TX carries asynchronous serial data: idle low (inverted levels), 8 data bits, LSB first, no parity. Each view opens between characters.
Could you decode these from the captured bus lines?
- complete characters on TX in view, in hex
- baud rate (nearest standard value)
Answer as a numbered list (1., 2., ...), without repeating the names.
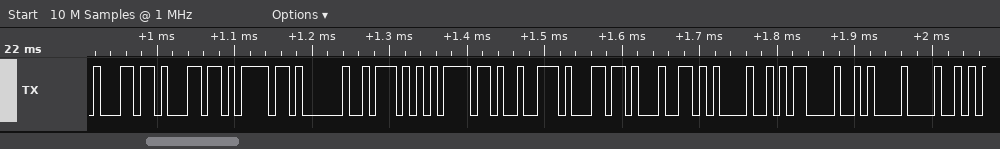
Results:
1. 27, 27, 21, BF, 51, 21, 1B, 27, 37, BD, E5, EB, 6F
2. 115200 baud
